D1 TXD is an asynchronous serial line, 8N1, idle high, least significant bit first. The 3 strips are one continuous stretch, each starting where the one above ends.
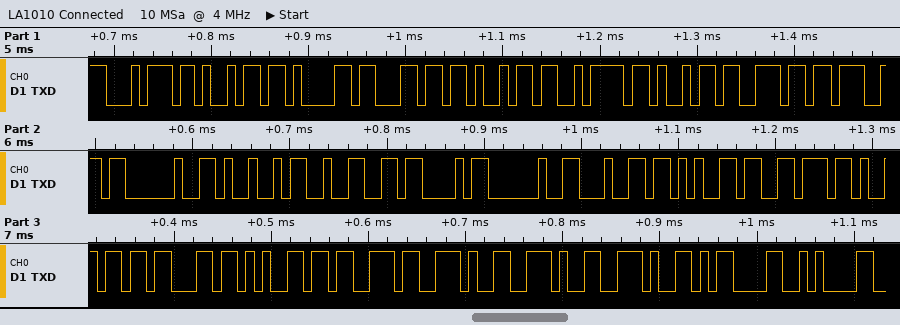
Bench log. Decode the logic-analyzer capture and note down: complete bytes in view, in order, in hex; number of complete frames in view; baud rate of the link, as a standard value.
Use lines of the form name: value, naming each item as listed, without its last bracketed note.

complete bytes in view, in order, in hex: 74 69 61 6C 69 7A 69 6E 67 20 49 32 43 20 64 65 76 69 63 65 73 2E 2E 2E 0D 0A
number of complete frames in view: 26
baud rate of the link, as a standard value: 115200 baud
